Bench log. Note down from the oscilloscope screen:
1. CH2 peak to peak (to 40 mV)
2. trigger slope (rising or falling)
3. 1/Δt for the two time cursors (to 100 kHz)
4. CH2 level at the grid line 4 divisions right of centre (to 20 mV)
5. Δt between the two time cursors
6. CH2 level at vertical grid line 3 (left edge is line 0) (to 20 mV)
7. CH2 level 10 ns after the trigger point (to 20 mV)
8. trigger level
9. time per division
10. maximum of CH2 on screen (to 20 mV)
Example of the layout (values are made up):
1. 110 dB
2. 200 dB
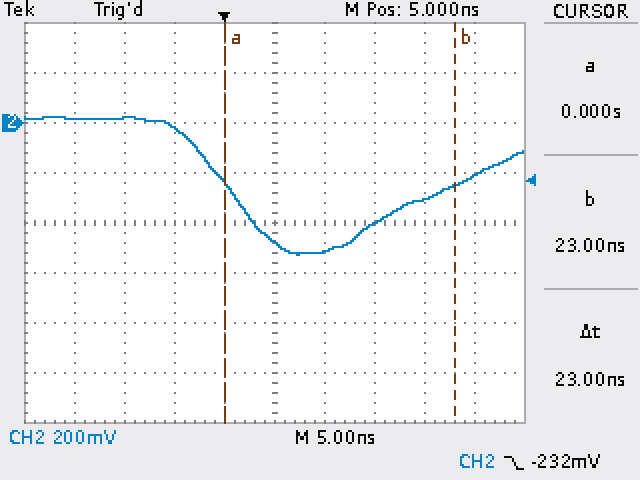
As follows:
1. 560 mV
2. falling
3. 43.5 MHz
4. -220 mV
5. 23 ns
6. -20 mV
7. -520 mV
8. -232 mV
9. 5 ns
10. 20 mV
